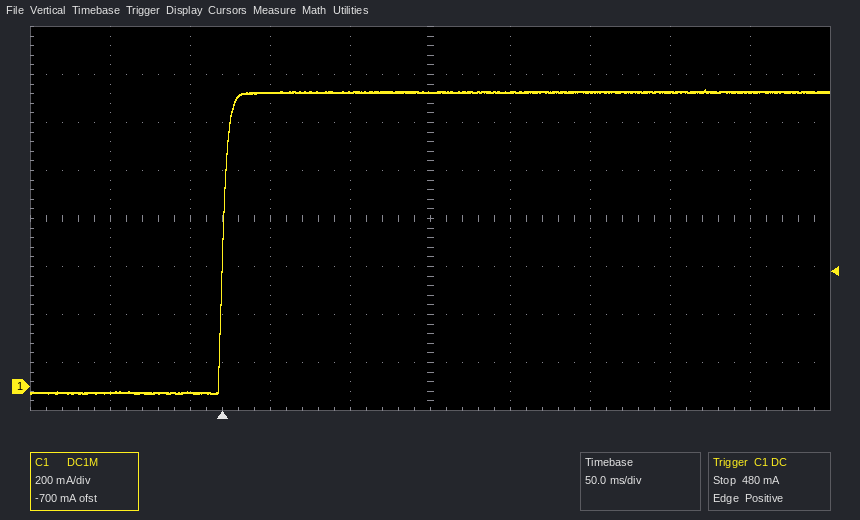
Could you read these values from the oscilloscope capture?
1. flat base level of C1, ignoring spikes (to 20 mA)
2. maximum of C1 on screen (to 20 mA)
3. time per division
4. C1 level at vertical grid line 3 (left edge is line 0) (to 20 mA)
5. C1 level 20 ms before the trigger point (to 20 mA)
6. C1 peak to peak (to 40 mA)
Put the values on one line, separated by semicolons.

-20 mA; 1.24 A; 50 ms; 1.22 A; -20 mA; 1.28 A
